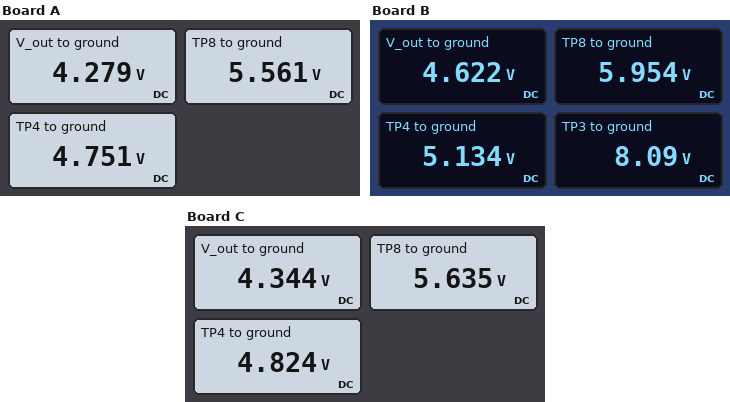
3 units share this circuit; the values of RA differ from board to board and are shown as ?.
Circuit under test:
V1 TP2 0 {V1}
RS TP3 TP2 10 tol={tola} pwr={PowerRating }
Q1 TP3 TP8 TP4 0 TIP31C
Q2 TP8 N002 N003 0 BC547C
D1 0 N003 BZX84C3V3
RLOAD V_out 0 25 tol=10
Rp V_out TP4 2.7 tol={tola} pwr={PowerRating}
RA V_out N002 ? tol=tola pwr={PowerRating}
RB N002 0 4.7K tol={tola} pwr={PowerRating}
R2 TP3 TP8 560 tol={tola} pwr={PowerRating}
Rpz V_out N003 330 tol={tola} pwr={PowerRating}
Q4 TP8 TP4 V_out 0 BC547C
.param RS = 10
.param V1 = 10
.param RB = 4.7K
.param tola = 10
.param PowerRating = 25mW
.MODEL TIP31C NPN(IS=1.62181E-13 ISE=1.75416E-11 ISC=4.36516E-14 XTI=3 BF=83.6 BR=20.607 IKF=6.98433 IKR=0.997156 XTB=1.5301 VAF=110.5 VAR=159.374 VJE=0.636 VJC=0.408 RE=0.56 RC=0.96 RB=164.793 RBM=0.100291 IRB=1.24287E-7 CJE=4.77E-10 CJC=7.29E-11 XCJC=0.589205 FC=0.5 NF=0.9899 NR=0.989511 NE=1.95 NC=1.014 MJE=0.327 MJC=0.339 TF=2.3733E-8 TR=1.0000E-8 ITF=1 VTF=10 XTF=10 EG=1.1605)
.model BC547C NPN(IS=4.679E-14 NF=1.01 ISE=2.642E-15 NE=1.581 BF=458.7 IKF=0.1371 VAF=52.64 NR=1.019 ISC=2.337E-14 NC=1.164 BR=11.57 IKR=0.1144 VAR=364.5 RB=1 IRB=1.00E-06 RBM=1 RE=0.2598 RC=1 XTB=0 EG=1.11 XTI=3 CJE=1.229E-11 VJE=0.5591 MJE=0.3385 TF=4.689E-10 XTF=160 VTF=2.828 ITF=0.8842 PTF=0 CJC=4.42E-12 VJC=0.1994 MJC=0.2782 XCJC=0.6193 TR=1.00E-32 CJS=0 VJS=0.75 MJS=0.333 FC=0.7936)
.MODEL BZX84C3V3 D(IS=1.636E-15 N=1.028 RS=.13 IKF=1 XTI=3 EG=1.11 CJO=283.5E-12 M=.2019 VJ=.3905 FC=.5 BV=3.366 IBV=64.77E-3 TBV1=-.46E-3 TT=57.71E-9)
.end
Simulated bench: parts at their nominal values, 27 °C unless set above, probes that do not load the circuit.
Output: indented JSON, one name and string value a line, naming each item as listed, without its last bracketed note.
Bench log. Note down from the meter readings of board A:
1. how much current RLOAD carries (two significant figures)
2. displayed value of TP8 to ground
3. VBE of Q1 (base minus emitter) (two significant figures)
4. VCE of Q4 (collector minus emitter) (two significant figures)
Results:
{
  "how much current RLOAD carries": "170 mA",
  "displayed value of TP8 to ground": "5.561 V",
  "VBE of Q1 (base minus emitter)": "810 mV",
  "VCE of Q4 (collector minus emitter)": "1.3 V"
}
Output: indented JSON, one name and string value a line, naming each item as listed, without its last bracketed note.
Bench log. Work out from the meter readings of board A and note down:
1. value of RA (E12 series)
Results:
{
  "value of RA": "390 Ω"
}
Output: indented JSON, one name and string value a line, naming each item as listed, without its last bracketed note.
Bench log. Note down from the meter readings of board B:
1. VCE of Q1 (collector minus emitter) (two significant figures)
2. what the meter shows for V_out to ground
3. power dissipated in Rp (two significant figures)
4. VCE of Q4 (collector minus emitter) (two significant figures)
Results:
{
  "VCE of Q1 (collector minus emitter)": "3.0 V",
  "what the meter shows for V_out to ground": "4.622 V",
  "power dissipated in Rp": "97 mW",
  "VCE of Q4 (collector minus emitter)": "1.3 V"
}
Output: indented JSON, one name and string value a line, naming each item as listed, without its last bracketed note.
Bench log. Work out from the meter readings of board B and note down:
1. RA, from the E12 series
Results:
{
  "RA, from the E12 series": "820 Ω"
}
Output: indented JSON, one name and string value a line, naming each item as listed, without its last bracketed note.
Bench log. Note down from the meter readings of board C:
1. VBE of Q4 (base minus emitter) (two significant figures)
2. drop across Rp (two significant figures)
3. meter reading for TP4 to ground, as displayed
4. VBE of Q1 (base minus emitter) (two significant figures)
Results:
{
  "VBE of Q4 (base minus emitter)": "480 mV",
  "drop across Rp": "480 mV",
  "meter reading for TP4 to ground, as displayed": "4.824 V",
  "VBE of Q1 (base minus emitter)": "810 mV"
}
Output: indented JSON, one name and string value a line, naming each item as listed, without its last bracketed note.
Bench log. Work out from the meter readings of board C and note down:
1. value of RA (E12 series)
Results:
{
  "value of RA": "470 Ω"
}
